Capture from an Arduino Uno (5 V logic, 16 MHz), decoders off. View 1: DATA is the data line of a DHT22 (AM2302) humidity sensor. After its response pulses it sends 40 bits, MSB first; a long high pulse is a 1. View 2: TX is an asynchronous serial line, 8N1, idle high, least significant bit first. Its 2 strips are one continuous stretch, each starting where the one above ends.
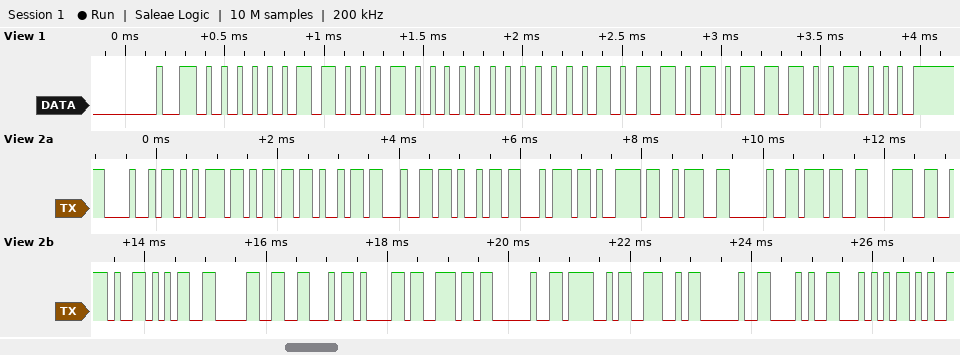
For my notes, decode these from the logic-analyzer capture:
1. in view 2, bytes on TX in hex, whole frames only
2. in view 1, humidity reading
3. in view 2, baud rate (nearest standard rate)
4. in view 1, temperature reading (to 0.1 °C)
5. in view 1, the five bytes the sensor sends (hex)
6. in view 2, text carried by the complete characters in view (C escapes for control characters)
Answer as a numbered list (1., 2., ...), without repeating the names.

1. 0x48 0x75 0x6D 0x69 0x64 0x69 0x74 0x79 0x3A 0x20 0x37 0x38 0x2E 0x35 0x30 0x46 0x61 0x6E 0x20 0x4F 0x4E 0x20 0x28 0x54
2. 78.4 %
3. 9600 baud
4. 18.1 °C
5. 03 10 00 B5 C8
6. "Humidity: 78.50Fan ON (T"
